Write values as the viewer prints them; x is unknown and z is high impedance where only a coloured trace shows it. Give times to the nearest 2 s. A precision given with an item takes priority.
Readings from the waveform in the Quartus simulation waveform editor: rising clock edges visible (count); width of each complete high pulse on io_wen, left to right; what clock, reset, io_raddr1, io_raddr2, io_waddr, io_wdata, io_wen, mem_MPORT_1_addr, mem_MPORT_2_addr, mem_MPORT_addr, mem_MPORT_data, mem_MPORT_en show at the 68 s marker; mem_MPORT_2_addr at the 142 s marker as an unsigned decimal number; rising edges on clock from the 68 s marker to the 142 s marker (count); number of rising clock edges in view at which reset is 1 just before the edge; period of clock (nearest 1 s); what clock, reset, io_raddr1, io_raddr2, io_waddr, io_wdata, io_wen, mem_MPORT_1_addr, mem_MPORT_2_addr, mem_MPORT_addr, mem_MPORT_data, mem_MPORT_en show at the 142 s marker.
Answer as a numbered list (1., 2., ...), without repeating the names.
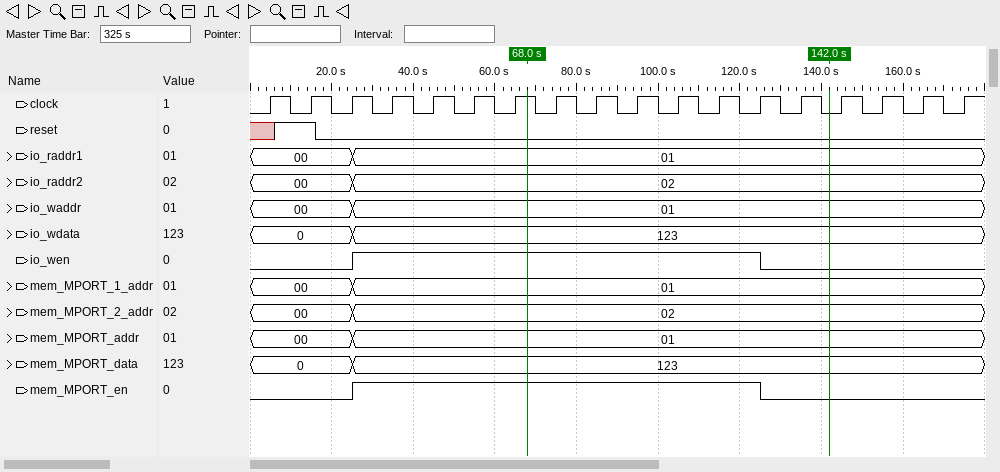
1. 18
2. 100 s
3. clock=1, reset=0, io_raddr1=01, io_raddr2=02, io_waddr=01, io_wdata=123, io_wen=1, mem_MPORT_1_addr=01, mem_MPORT_2_addr=02, mem_MPORT_addr=01, mem_MPORT_data=123, mem_MPORT_en=1
4. 2
5. 7
6. 1
7. 10 s
8. clock=0, reset=0, io_raddr1=01, io_raddr2=02, io_waddr=01, io_wdata=123, io_wen=0, mem_MPORT_1_addr=01, mem_MPORT_2_addr=02, mem_MPORT_addr=01, mem_MPORT_data=123, mem_MPORT_en=0
